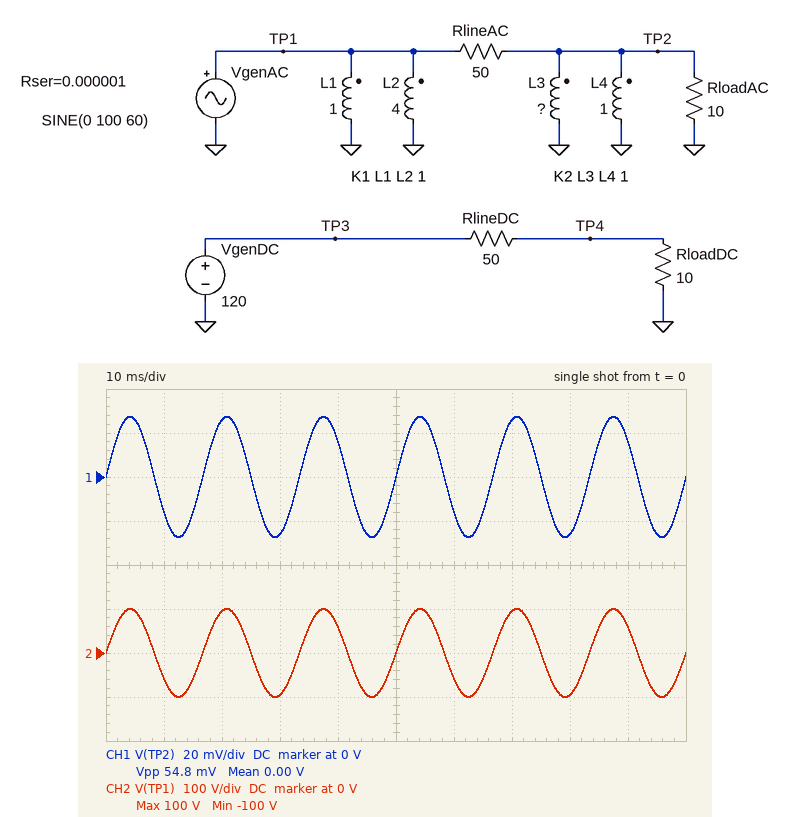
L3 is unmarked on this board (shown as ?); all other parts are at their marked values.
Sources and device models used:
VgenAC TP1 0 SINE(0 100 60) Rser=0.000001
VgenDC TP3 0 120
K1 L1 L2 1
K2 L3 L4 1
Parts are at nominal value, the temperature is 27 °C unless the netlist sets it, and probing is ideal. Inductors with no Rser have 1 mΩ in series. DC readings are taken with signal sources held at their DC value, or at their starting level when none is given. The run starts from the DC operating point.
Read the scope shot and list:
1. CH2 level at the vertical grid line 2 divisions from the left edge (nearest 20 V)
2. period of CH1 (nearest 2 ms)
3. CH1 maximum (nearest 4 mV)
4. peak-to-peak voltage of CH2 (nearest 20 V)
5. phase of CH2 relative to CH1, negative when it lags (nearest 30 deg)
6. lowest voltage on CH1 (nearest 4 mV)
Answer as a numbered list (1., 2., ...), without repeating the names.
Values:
1. 100 V
2. 16 ms
3. 28 mV
4. 200 V
5. 0 deg
6. -28 mV
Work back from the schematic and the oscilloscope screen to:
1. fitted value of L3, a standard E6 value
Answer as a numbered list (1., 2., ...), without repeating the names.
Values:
1. 2.2 H
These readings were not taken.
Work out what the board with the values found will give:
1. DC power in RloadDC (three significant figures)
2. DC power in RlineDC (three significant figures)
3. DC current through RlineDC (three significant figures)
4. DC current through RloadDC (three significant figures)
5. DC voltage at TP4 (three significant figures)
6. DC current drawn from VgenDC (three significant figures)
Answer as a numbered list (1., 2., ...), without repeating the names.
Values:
1. 40.0 W
2. 200 W
3. 2.00 A
4. 2.00 A
5. 20.0 V
6. 2.00 A
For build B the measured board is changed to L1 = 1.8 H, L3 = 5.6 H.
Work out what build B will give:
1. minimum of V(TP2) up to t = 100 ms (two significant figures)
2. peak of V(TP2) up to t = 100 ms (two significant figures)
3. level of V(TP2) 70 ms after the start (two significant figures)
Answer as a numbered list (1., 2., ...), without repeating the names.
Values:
1. -7.1 mV
2. 7.1 mV
3. 6.7 mV
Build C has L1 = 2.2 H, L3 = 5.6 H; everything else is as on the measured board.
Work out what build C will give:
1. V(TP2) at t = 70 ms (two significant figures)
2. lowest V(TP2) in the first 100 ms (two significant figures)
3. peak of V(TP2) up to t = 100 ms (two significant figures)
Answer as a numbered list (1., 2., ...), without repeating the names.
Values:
1. 6.7 mV
2. -7.1 mV
3. 7.1 mV
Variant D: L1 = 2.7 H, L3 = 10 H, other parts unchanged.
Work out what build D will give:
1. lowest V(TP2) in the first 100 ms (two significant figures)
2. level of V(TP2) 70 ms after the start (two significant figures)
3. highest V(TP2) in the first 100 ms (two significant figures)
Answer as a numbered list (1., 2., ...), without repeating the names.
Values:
1. -4.7 mV
2. 4.5 mV
3. 4.7 mV
